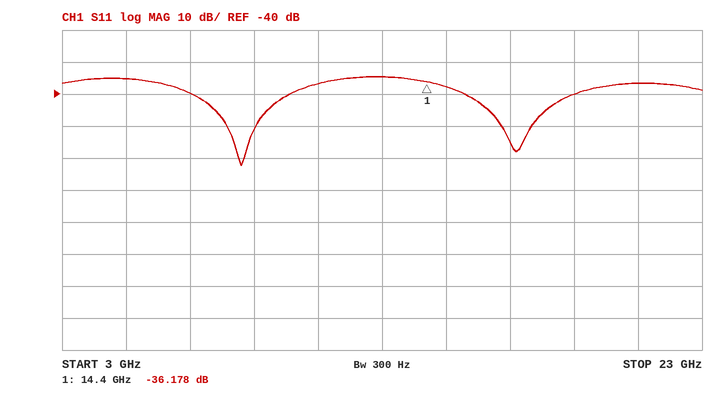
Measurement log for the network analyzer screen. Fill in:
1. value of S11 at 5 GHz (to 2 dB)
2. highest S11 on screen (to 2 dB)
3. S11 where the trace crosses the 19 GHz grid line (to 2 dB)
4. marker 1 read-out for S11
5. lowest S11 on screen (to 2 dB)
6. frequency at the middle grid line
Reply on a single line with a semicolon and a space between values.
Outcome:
-36 dB; -34 dB; -40 dB; -36.178 dB; -62 dB; 13 GHz
